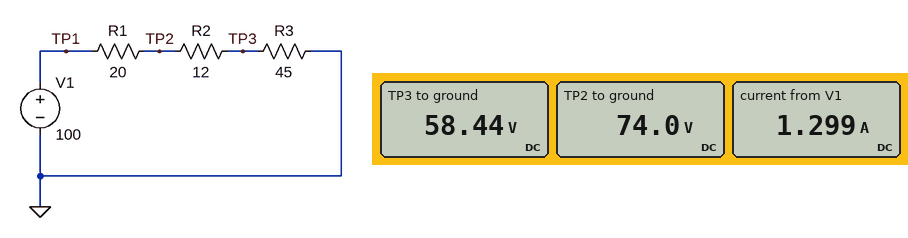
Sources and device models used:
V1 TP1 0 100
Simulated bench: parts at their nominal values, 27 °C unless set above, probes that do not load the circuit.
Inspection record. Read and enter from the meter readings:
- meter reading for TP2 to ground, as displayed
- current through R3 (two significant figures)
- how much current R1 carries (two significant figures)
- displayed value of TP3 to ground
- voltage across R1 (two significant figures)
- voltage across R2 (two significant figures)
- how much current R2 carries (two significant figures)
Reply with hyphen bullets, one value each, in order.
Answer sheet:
- 74.0 V
- 1.3 A
- 1.3 A
- 58.44 V
- 26 V
- 16 V
- 1.3 A
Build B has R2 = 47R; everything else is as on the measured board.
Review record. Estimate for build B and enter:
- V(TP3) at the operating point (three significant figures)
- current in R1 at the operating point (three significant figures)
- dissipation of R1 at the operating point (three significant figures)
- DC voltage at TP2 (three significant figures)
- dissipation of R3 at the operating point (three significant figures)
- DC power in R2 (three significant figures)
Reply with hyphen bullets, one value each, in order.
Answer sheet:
- 40.2 V
- 893 mA
- 15.9 W
- 82.1 V
- 35.9 W
- 37.5 W
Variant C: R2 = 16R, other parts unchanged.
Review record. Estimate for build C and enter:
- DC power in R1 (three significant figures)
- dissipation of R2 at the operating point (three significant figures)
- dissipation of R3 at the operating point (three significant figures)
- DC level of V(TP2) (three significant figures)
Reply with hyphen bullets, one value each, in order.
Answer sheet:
- 30.5 W
- 24.4 W
- 68.6 W
- 75.3 V
